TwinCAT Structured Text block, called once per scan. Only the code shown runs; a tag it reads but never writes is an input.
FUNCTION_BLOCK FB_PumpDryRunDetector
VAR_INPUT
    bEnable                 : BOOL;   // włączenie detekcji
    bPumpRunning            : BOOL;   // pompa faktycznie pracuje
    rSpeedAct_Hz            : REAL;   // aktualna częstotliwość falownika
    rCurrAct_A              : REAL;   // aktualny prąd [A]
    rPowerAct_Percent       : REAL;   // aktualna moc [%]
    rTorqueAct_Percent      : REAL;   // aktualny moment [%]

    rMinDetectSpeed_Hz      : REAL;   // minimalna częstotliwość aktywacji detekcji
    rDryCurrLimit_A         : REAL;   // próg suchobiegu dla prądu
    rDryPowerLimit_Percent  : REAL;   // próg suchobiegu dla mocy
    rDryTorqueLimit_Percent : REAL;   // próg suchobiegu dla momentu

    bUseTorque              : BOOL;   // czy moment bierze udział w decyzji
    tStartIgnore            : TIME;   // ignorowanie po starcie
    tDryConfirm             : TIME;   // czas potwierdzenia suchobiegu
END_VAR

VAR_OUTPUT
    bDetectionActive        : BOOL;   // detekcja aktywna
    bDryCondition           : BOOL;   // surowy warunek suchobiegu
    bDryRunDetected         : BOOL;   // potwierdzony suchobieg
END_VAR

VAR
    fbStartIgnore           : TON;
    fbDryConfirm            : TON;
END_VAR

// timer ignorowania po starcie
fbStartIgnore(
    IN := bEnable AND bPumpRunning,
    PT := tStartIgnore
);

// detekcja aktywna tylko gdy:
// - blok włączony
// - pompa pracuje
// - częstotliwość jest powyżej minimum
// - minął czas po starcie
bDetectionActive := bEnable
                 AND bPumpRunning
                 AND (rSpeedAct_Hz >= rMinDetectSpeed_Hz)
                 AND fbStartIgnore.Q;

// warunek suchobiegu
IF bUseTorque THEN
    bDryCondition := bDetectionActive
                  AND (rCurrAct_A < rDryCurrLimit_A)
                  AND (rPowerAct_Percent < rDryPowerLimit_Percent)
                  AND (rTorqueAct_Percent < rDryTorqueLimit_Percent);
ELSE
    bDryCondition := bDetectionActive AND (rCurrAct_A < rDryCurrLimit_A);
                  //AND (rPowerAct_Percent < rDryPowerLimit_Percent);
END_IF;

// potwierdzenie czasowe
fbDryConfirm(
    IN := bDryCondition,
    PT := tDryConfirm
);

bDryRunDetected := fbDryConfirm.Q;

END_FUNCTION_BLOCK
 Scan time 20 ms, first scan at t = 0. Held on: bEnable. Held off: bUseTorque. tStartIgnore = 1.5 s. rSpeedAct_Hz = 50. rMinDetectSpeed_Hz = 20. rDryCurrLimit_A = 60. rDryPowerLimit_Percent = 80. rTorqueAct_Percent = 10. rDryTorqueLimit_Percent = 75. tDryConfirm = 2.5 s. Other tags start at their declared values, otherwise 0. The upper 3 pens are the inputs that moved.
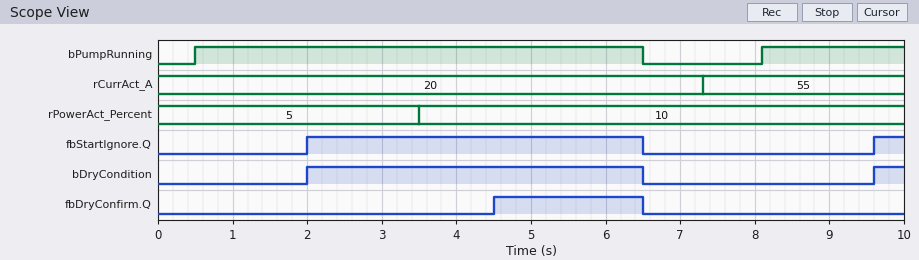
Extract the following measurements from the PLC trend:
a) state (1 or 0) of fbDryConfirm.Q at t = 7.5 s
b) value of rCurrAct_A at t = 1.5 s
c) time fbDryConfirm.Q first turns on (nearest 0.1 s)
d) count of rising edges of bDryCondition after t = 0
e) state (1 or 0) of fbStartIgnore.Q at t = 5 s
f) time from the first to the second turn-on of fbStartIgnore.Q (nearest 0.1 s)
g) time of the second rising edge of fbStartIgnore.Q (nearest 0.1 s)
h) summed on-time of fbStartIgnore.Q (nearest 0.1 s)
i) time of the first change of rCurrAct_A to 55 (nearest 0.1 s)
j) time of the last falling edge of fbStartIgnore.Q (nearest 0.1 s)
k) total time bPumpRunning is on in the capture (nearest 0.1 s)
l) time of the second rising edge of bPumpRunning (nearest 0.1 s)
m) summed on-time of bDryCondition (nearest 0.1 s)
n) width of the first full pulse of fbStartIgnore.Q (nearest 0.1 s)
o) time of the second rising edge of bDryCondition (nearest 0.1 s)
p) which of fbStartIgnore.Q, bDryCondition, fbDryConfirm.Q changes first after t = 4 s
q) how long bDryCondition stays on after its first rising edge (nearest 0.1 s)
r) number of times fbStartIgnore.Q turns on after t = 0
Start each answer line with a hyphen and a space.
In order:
- 0
- 20
- 4.5 s
- 2
- 1
- 7.6 s
- 9.6 s
- 4.9 s
- 7.3 s
- 6.5 s
- 7.9 s
- 8.1 s
- 4.9 s
- 4.5 s
- 9.6 s
- fbDryConfirm.Q
- 4.5 s
- 2
